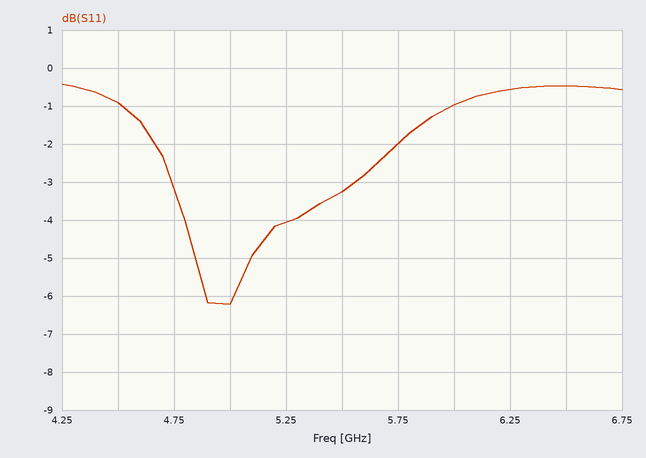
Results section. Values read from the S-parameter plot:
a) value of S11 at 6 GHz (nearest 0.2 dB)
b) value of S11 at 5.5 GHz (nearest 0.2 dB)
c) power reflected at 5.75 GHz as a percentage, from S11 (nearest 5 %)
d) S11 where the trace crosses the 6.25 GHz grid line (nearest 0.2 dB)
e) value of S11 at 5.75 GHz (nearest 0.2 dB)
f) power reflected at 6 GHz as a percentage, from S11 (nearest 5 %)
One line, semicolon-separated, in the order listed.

-1.0 dB; -3.2 dB; 65 %; -0.6 dB; -2.0 dB; 80 %
